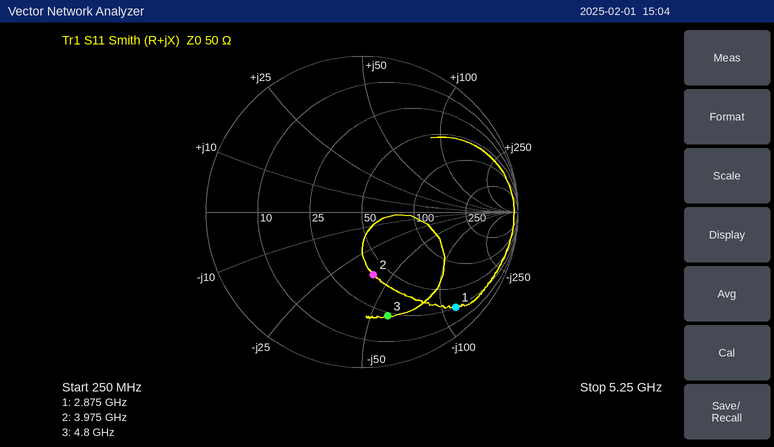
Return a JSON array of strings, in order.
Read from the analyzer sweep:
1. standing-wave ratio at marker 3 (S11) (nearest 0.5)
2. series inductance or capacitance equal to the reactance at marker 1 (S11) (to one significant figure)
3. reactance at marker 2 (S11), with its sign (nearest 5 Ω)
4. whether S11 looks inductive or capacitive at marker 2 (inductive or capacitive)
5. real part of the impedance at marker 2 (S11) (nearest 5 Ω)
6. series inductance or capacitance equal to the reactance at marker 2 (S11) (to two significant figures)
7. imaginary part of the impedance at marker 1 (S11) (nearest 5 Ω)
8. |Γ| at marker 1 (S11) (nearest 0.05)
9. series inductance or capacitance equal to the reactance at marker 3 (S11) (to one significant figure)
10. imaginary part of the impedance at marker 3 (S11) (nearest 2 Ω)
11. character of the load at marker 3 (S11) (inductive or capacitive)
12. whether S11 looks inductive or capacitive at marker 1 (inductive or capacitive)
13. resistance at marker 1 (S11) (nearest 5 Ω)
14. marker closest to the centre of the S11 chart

["5.5", "500 fF", "-40 Ω", "capacitive", "40 Ω", "1.0 pF", "-115 Ω", "0.85", "600 fF", "-58 Ω", "capacitive", "capacitive", "25 Ω", "marker 2"]
